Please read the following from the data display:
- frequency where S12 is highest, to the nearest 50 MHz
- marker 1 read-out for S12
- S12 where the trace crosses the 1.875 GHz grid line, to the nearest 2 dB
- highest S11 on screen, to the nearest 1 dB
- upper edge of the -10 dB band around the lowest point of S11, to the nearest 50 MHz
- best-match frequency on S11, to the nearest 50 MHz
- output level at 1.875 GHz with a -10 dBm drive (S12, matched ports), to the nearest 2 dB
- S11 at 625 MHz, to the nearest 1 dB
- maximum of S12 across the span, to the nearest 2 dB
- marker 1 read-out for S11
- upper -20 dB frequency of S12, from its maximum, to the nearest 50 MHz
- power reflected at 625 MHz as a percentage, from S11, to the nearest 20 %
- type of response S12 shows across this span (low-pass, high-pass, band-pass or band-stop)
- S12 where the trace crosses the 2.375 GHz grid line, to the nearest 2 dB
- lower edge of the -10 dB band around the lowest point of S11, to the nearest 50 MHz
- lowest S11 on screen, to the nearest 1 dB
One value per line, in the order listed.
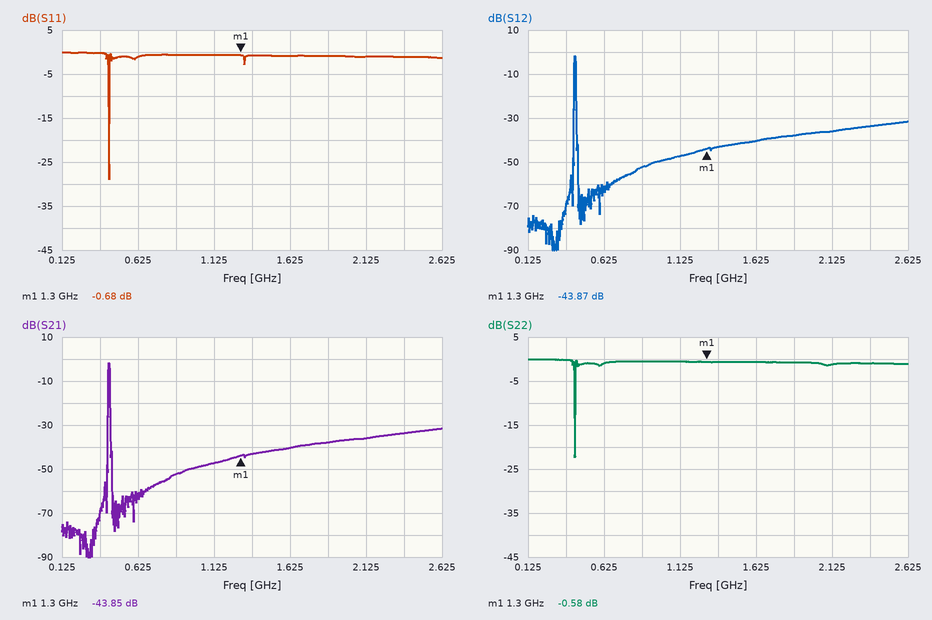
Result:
450 MHz
-43.87 dB
-38 dB
0 dB
450 MHz
450 MHz
-48 dBm
-1 dB
-2 dB
-0.68 dB
450 MHz
80 %
band-pass
-34 dB
450 MHz
-29 dB
